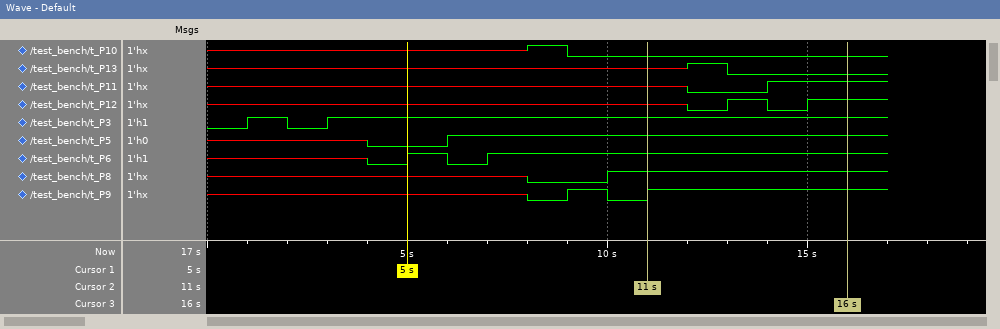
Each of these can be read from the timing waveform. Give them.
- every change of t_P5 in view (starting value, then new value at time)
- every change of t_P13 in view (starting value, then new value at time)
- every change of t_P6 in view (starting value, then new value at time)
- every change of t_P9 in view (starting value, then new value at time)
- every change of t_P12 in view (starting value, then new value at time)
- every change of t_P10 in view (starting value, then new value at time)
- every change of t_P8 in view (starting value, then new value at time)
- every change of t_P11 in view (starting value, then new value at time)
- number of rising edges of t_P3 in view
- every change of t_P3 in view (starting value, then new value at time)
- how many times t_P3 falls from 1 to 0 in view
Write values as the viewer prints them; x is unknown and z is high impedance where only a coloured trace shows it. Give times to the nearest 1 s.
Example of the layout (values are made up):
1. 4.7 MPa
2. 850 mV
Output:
1. x, 0 at 4 s, 1 at 6 s
2. x, 1 at 12 s, 0 at 13 s
3. x, 0 at 4 s, 1 at 5 s, 0 at 6 s, 1 at 7 s
4. x, 0 at 8 s, 1 at 9 s, 0 at 10 s, 1 at 11 s
5. x, 0 at 12 s, 1 at 13 s, 0 at 14 s, 1 at 15 s
6. x, 1 at 8 s, 0 at 9 s
7. x, 0 at 8 s, 1 at 10 s
8. x, 0 at 12 s, 1 at 14 s
9. 2
10. 0, 1 at 1 s, 0 at 2 s, 1 at 3 s
11. 1
